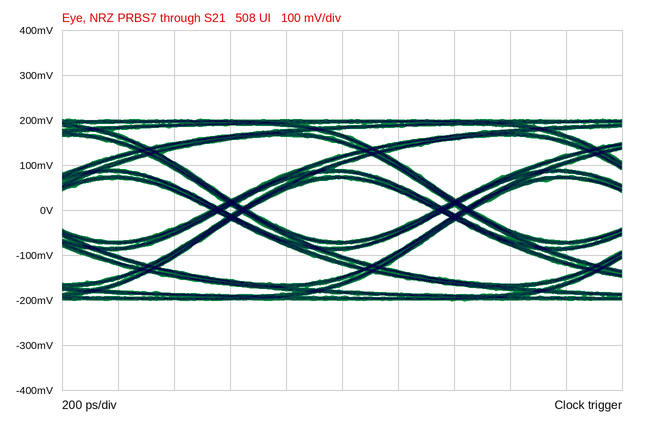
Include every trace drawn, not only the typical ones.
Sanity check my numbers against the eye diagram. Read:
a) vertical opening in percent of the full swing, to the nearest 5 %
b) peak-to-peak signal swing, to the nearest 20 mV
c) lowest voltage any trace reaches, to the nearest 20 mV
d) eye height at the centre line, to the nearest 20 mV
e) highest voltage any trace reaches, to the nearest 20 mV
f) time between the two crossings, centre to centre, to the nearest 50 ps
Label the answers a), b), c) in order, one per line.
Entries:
a) 35 %
b) 400 mV
c) -200 mV
d) 140 mV
e) 200 mV
f) 800 ps
